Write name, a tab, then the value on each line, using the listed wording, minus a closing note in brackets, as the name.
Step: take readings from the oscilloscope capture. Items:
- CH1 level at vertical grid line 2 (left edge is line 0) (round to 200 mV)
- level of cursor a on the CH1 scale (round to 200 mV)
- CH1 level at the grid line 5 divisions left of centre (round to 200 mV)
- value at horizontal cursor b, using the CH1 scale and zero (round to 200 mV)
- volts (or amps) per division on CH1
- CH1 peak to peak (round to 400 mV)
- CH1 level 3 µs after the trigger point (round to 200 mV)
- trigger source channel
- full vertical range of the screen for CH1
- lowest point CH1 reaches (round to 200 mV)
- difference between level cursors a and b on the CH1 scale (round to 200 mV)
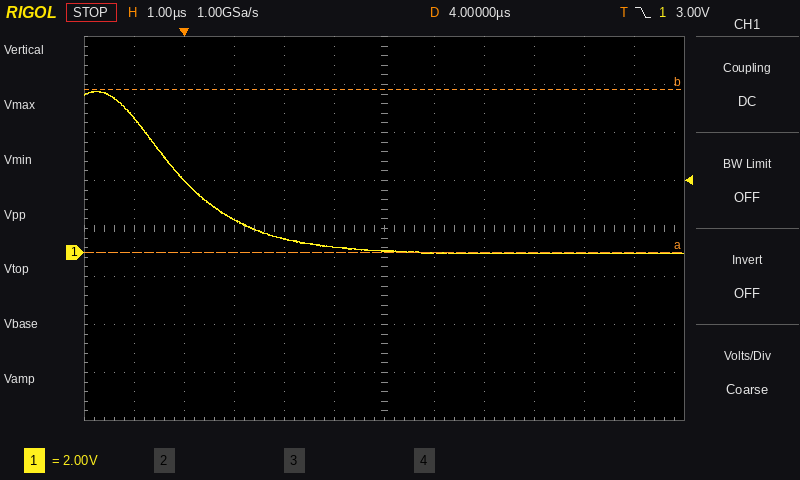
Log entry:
CH1 level at vertical grid line 2 (left edge is line 0)	3.0 V
level of cursor a on the CH1 scale	0.0 V
CH1 level at the grid line 5 divisions left of centre	5.6 V
value at horizontal cursor b, using the CH1 scale and zero	6.8 V
volts (or amps) per division on CH1	2 V
CH1 peak to peak	6.8 V
CH1 level 3 µs after the trigger point	200 mV
trigger source channel	CH1
full vertical range of the screen for CH1	16 V
lowest point CH1 reaches	0.0 V
difference between level cursors a and b on the CH1 scale	6.8 V
